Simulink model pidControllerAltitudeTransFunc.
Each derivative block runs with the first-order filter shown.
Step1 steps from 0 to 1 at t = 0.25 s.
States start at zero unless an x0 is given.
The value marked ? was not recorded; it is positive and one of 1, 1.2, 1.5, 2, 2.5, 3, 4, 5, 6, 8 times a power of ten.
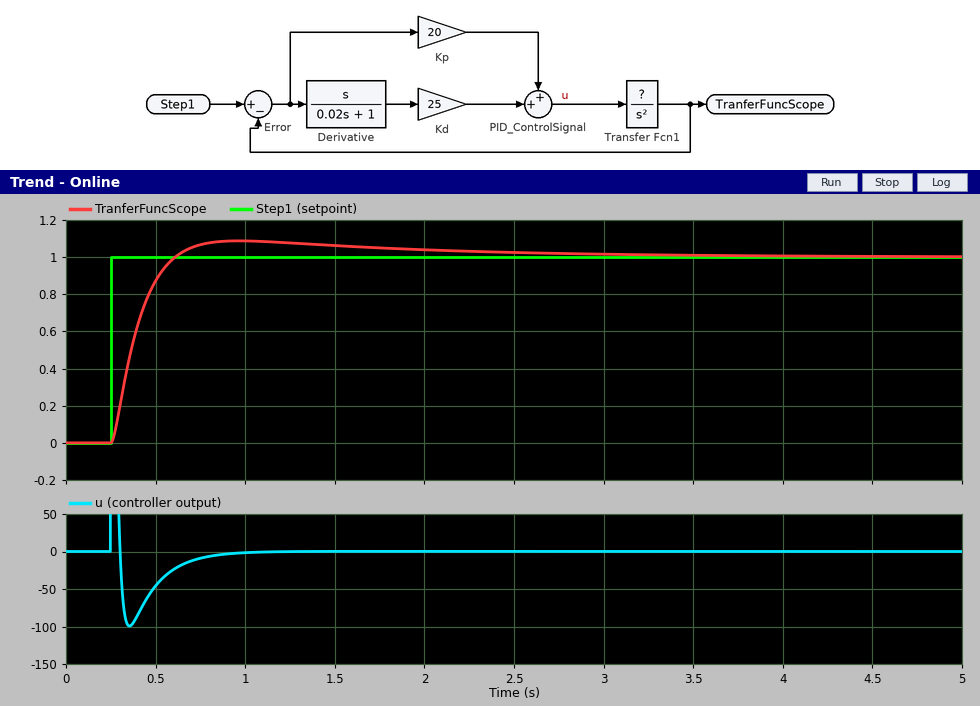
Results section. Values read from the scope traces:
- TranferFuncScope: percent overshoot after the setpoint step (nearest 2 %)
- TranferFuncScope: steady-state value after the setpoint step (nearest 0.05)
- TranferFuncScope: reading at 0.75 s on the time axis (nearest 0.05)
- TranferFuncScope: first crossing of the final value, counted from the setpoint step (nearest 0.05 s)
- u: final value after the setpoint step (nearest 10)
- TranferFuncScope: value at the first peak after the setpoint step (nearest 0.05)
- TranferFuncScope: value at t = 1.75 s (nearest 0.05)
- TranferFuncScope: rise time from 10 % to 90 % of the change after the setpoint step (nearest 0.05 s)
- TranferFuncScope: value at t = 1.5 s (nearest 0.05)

8 %
1.00
1.05
0.35 s
0
1.10
1.05
0.25 s
1.05
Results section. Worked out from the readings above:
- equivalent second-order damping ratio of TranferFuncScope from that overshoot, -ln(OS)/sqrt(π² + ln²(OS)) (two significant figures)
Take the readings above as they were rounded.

0.63
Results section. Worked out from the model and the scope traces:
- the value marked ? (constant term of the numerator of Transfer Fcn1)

0.25
